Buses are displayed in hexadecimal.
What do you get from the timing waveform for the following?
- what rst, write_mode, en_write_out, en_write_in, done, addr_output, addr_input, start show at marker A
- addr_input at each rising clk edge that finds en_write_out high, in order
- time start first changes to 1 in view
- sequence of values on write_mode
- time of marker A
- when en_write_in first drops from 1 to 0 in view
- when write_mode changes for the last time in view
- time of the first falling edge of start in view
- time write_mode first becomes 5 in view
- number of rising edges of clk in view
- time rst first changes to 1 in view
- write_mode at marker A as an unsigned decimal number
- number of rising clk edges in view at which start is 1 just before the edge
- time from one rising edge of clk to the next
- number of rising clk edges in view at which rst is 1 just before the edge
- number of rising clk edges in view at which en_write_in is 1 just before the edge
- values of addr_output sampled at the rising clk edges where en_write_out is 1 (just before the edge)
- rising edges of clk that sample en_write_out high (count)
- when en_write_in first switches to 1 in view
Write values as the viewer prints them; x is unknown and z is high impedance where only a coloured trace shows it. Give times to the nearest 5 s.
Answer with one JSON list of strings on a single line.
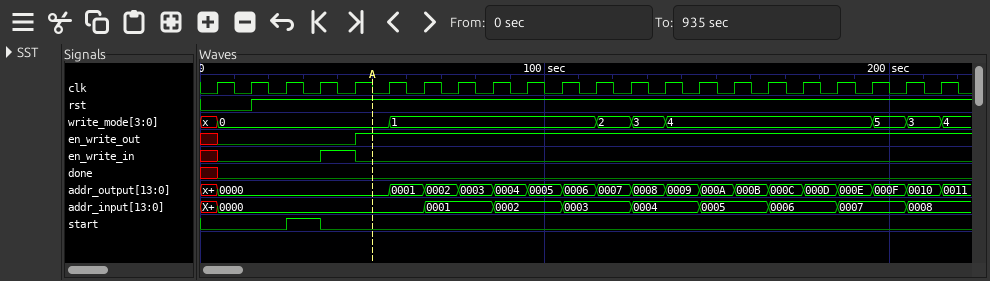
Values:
["rst=1, write_mode=0, en_write_out=1, en_write_in=0, done=0, addr_output=0000, addr_input=0000, start=0", "0000, 0000, 0001, 0001, 0002, 0002, 0003, 0003, 0004, 0004, 0005, 0005, 0006, 0006, 0007, 0007, 0008", "25 s", "x, 0, 1, 2, 3, 4, 5, 3, 4", "50 s", "45 s", "215 s", "35 s", "195 s", "22", "15 s", "0", "1", "10 s", "20", "1", "0000, 0001, 0002, 0003, 0004, 0005, 0006, 0007, 0008, 0009, 000A, 000B, 000C, 000D, 000E, 000F, 0010", "17", "35 s"]
